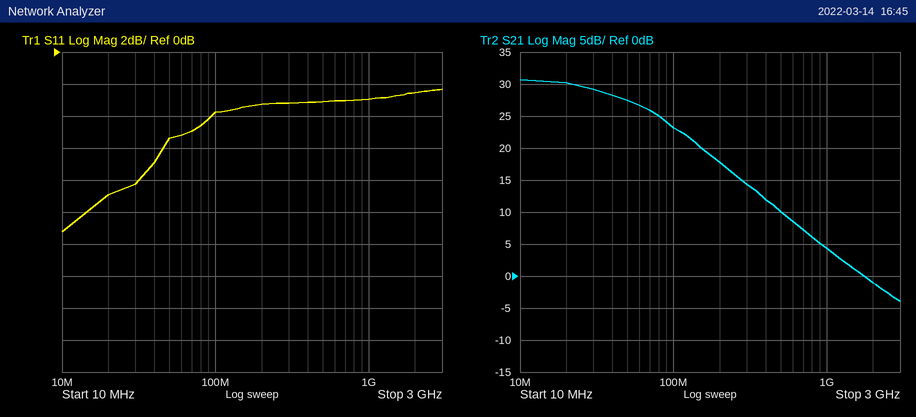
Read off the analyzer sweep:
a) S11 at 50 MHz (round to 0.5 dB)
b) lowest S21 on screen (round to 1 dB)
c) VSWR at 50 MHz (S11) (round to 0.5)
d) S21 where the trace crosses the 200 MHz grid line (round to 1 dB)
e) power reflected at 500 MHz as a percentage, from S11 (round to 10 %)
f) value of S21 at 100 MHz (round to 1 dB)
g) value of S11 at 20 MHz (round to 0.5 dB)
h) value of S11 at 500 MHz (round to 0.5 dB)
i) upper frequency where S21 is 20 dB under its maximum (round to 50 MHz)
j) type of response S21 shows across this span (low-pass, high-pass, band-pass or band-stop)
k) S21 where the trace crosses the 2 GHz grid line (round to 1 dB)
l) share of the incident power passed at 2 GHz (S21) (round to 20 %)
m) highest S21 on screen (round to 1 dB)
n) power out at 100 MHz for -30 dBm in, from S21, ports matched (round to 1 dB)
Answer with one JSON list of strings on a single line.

["-5.5 dB", "-4 dB", "3.5", "18 dB", "50 %", "23 dB", "-9.0 dB", "-3.0 dB", "450 MHz", "low-pass", "-1 dB", "80 %", "31 dB", "-7 dBm"]
